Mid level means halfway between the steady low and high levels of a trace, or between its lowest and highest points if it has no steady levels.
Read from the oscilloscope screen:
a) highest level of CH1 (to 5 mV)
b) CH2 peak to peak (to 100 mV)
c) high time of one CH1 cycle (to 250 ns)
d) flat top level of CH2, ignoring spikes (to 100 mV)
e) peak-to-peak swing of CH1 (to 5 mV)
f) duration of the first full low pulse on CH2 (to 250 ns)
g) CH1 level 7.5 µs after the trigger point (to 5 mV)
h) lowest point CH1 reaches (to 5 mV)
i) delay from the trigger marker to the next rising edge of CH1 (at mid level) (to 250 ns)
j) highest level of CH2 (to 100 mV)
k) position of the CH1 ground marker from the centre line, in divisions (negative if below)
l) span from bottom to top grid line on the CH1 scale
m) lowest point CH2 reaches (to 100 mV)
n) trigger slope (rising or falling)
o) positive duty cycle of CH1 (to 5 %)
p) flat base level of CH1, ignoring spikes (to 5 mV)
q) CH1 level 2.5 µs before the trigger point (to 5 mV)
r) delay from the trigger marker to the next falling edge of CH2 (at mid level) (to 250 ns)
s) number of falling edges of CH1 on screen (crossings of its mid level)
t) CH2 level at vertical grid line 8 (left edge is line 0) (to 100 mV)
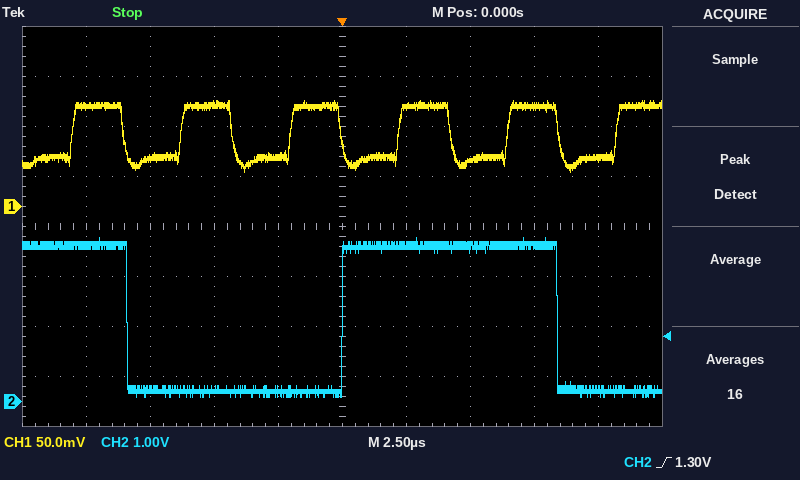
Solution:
105 mV
3.2 V
2.00 µs
3.1 V
70 mV
8.50 µs
100 mV
35 mV
2.25 µs
3.3 V
+0.4 div
400 mV
100 mV
rising
45 %
50 mV
50 mV
8.50 µs
5
3.1 V
